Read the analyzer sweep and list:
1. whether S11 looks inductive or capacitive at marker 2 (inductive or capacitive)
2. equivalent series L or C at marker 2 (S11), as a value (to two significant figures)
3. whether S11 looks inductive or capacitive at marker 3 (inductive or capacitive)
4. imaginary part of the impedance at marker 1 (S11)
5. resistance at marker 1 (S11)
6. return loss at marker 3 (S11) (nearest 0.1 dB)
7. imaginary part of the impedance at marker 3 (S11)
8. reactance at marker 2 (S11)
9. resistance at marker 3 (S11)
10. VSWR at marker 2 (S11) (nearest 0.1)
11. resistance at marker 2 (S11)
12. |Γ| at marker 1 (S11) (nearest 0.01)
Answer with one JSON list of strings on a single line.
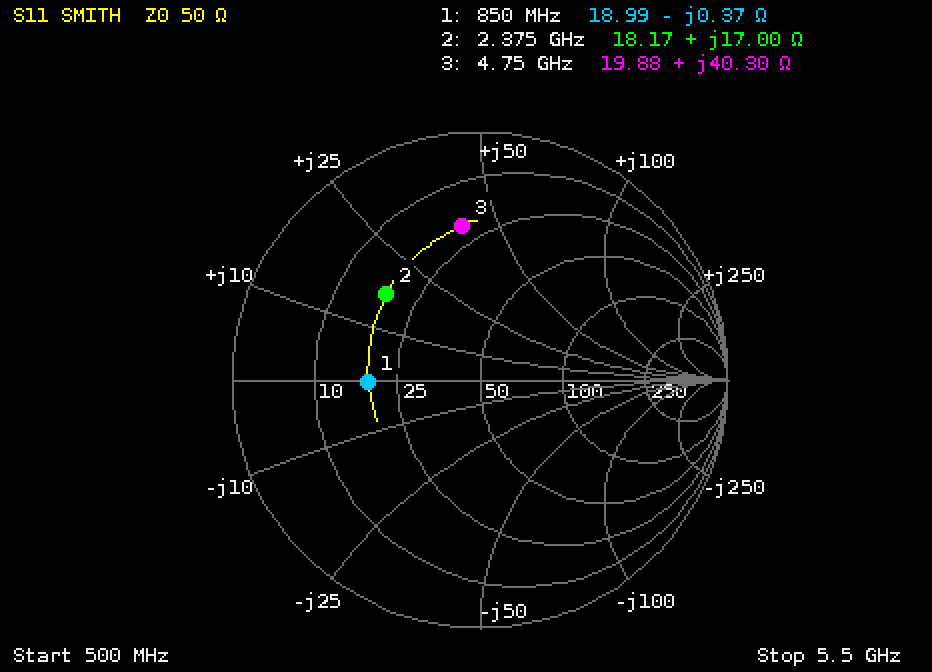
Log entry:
["inductive", "1.1 nH", "inductive", "-0.37 Ω", "18.99 Ω", "4.1 dB", "+40.30 Ω", "+17.00 Ω", "19.88 Ω", "3.1", "18.17 Ω", "0.45"]
